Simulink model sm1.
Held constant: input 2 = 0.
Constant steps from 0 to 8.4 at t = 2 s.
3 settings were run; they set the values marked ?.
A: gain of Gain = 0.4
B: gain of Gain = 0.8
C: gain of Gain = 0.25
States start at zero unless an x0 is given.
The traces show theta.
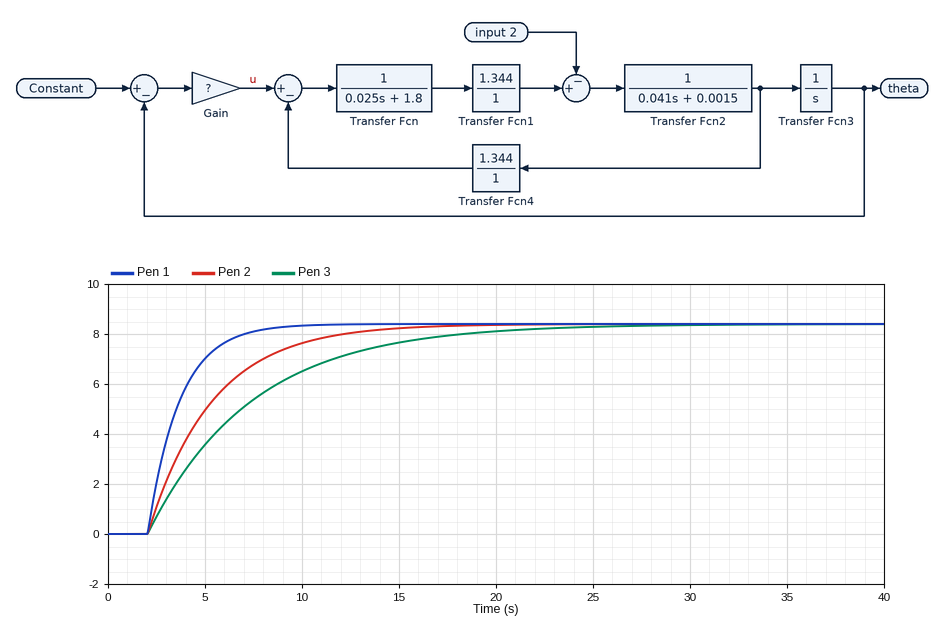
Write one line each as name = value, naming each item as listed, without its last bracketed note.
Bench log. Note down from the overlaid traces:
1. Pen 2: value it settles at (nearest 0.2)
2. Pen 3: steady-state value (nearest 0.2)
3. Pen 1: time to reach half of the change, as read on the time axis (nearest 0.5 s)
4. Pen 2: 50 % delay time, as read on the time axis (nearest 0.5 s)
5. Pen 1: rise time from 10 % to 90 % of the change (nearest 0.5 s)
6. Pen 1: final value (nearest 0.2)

Pen 2: value it settles at = 8.4
Pen 3: steady-state value = 8.4
Pen 1: time to reach half of the change, as read on the time axis = 3.0 s
Pen 2: 50 % delay time, as read on the time axis = 4.5 s
Pen 1: rise time from 10 % to 90 % of the change = 3.5 s
Pen 1: final value = 8.4
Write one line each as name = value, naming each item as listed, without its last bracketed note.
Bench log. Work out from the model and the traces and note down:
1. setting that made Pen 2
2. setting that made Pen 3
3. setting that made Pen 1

setting that made Pen 2 = A
setting that made Pen 3 = C
setting that made Pen 1 = B
